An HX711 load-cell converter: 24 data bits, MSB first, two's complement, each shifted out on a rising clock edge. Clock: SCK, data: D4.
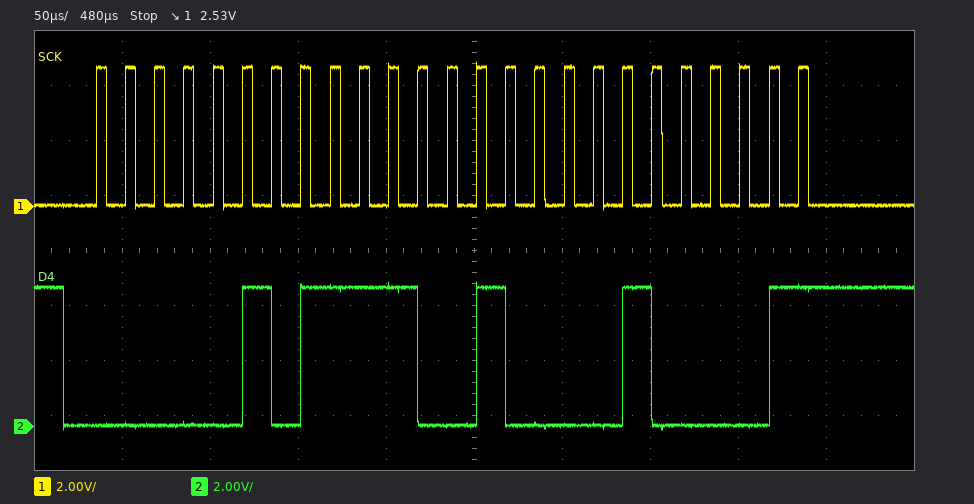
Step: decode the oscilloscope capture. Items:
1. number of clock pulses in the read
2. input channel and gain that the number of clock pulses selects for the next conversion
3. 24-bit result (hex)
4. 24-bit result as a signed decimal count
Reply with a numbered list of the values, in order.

1. 25
2. channel A, gain 128
3. 0x05E421
4. 386081
